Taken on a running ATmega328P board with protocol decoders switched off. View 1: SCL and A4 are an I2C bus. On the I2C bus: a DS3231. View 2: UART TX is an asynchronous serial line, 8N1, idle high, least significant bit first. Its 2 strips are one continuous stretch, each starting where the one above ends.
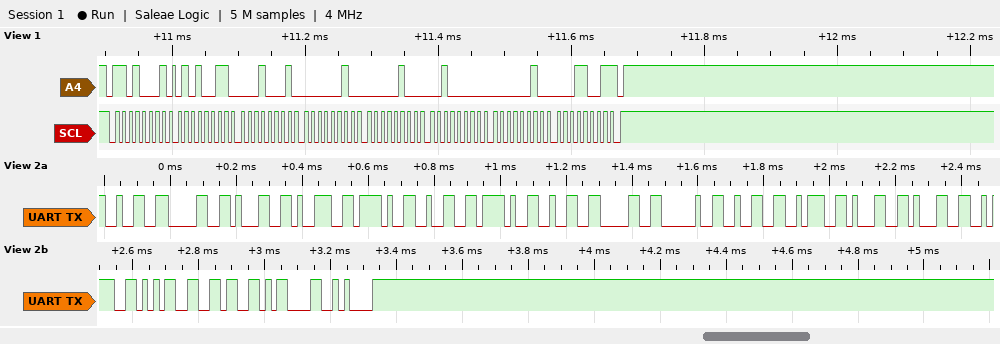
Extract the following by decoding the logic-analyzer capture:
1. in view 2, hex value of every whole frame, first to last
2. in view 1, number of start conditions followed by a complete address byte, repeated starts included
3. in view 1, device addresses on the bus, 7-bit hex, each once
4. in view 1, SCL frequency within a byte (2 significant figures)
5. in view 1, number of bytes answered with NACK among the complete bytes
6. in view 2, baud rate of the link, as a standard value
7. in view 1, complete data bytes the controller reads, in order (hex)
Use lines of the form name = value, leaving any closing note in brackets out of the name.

in view 2, hex value of every whole frame, first to last = 0x32 0x30 0x31 0x39 0x2F 0x32 0x2F 0x32 0x30 0x20 0x32 0x3A 0x31 0x31 0x3A 0x35 0x36 0x0D 0x0A
in view 1, number of start conditions followed by a complete address byte, repeated starts included = 1
in view 1, device addresses on the bus, 7-bit hex, each once = 0x68
in view 1, SCL frequency within a byte = 100 kHz
in view 1, number of bytes answered with NACK among the complete bytes = 1
in view 2, baud rate of the link, as a standard value = 57600 baud
in view 1, complete data bytes the controller reads, in order = 53 11 02 04 20 02 19
